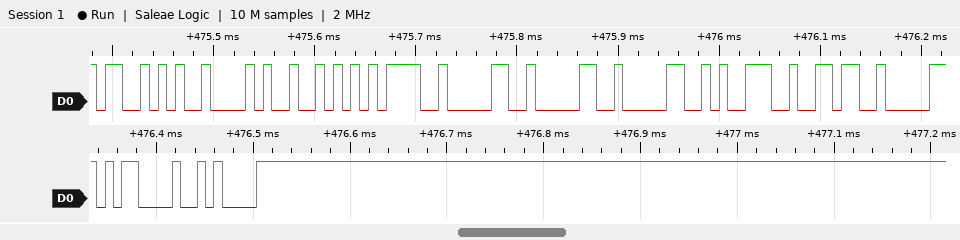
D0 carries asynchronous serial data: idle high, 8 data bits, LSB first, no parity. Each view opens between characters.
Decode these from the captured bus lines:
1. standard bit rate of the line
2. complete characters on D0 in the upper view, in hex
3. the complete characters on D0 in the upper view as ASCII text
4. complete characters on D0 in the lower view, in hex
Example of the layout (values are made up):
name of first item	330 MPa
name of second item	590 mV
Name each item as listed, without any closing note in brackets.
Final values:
standard bit rate of the line	115200 baud
complete characters on D0 in the upper view, in hex	53, 42, 52, 3D, 30, 30, 30, 39, 36
the complete characters on D0 in the upper view as ASCII text	"SBR=00096"
complete characters on D0 in the lower view, in hex	0D, 0A
